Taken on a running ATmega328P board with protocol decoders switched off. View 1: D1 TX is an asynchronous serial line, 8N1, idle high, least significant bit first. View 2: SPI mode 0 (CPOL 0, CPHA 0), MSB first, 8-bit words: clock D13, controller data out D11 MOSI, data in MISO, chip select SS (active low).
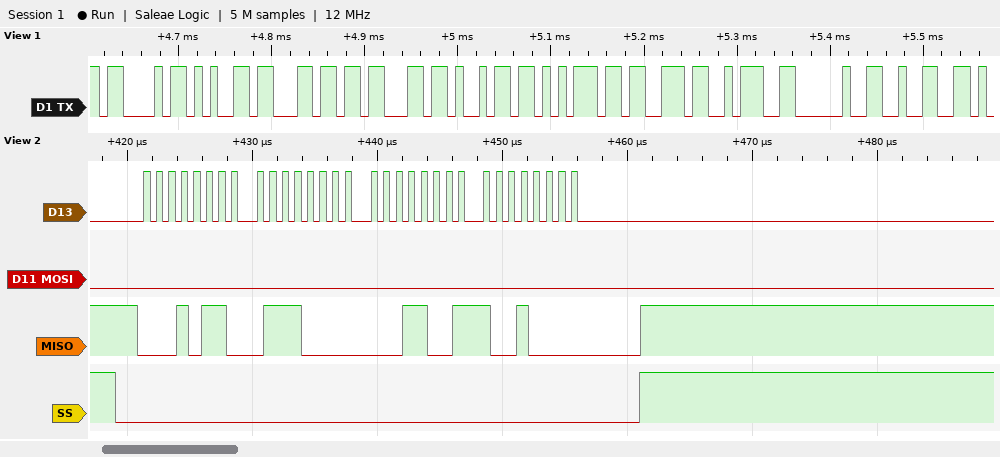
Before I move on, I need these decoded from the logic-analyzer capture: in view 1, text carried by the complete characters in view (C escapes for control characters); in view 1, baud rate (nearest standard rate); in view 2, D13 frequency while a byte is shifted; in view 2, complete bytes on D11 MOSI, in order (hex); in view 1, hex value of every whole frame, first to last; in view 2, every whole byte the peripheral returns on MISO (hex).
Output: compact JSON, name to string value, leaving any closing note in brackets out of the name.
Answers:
{"in view 1, text carried by the complete characters in view": "\"Celcius: 2\"", "in view 1, baud rate": "115200 baud", "in view 2, D13 frequency while a byte is shifted": "1 MHz", "in view 2, complete bytes on D11 MOSI, in order": "00 00 00 00", "in view 1, hex value of every whole frame, first to last": "43 65 6C 63 69 75 73 3A 20 32", "in view 2, every whole byte the peripheral returns on MISO": "16 70 19 90"}
